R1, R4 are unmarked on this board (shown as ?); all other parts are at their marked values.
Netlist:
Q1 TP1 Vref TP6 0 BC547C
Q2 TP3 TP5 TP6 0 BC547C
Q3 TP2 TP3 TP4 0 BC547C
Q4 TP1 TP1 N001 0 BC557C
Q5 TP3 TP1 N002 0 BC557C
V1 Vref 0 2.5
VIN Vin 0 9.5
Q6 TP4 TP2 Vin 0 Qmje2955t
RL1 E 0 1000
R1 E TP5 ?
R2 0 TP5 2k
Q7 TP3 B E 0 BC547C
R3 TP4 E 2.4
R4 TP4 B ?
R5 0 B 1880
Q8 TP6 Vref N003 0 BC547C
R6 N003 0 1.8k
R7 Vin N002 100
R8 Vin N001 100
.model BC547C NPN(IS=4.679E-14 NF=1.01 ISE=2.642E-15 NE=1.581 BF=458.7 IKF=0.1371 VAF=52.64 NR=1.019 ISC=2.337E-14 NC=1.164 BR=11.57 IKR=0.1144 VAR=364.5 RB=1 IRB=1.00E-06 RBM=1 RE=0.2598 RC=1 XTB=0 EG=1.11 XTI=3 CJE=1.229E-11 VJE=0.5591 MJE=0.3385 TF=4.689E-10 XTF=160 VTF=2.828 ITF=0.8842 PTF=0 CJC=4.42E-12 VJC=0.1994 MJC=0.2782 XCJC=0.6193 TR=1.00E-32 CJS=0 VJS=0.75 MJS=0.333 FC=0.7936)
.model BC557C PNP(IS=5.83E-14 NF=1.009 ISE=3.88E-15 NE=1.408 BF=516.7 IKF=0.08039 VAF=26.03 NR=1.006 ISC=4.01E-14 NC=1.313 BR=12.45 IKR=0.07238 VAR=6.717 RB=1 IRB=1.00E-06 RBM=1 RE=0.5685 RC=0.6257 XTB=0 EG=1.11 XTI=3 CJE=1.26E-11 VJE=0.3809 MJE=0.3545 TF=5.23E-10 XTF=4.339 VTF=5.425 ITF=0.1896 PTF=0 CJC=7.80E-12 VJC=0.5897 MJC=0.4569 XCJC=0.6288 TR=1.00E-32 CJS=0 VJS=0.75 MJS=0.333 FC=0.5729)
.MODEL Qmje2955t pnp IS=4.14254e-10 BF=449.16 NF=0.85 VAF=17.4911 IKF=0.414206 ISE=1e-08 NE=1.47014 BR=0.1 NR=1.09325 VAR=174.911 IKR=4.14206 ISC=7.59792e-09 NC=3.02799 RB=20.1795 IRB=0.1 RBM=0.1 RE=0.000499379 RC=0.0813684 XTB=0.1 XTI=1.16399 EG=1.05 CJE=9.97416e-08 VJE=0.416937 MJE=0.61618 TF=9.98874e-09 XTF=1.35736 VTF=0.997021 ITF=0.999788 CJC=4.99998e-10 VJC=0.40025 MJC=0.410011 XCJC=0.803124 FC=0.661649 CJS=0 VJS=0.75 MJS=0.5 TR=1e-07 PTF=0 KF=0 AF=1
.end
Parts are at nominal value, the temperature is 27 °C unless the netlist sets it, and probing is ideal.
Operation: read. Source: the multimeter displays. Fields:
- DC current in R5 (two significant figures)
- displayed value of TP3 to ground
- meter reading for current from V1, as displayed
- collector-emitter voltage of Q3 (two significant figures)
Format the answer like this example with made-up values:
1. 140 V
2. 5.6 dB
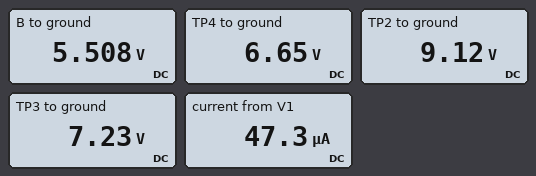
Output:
1. 2.9 mA
2. 7.23 V
3. 47.3 µA
4. 2.5 V
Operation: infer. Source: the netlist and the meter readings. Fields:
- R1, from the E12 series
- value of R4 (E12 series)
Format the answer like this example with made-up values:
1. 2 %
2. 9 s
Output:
1. 3.3 kΩ
2. 390 Ω
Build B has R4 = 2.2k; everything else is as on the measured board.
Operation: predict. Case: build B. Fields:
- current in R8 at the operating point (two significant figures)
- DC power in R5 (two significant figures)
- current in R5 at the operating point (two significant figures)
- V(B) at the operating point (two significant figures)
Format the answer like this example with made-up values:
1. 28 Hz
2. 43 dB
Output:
1. 490 µA
2. 5.0 mW
3. 1.6 mA
4. 3.1 V
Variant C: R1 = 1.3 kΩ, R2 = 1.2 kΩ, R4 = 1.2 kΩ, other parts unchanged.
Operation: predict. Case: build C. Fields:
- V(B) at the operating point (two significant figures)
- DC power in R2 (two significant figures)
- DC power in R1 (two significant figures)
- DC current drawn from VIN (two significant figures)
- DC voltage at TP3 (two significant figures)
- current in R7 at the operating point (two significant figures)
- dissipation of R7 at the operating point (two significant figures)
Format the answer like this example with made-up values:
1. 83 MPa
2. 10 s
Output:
1. 3.2 V
2. 5.2 mW
3. 5.7 mW
4. 10 mA
5. 5.8 V
6. 510 µA
7. 26 µW
